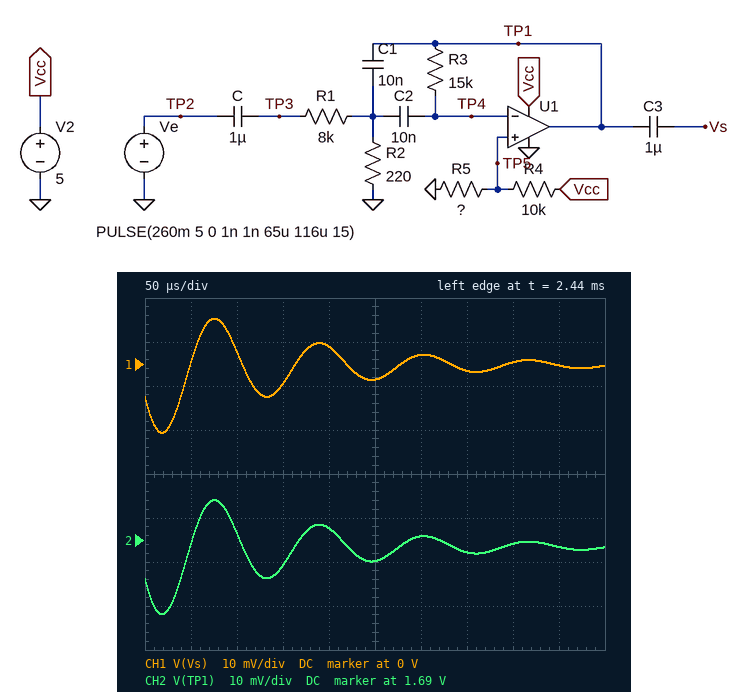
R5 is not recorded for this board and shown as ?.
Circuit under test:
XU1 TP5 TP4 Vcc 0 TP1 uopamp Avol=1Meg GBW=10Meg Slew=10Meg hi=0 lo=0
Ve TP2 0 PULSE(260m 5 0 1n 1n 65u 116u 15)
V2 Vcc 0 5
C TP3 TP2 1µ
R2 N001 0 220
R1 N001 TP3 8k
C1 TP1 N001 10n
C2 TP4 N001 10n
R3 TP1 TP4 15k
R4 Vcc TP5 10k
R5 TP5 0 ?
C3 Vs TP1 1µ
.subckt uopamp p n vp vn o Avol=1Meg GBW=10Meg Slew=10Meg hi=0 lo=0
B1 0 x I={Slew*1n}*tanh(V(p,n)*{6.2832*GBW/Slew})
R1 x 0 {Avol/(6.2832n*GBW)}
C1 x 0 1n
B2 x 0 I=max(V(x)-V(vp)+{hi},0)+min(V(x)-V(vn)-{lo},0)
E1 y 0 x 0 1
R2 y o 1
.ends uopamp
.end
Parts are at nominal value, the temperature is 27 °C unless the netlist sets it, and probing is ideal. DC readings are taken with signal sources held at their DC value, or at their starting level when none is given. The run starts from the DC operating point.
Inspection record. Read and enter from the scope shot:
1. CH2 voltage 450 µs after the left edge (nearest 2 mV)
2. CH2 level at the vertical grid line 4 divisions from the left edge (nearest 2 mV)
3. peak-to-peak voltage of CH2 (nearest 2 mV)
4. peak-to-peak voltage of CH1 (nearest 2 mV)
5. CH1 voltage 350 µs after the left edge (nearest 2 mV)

1.688 V
1.692 V
26 mV
26 mV
-2 mV
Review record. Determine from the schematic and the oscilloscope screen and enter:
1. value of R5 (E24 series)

5.1 kΩ
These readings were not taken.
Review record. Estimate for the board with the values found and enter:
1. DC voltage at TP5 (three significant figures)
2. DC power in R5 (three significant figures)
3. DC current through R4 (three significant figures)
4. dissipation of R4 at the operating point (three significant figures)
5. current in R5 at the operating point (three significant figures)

1.69 V
559 µW
331 µA
1.10 mW
331 µA
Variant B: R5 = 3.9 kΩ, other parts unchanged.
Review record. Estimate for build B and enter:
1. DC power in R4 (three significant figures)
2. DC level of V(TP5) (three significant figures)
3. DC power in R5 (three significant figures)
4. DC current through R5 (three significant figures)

1.29 mW
1.40 V
505 µW
360 µA
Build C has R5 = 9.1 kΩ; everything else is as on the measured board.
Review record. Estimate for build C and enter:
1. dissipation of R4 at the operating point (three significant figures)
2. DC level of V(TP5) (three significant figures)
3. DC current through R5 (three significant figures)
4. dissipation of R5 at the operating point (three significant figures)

685 µW
2.38 V
262 µA
624 µW
